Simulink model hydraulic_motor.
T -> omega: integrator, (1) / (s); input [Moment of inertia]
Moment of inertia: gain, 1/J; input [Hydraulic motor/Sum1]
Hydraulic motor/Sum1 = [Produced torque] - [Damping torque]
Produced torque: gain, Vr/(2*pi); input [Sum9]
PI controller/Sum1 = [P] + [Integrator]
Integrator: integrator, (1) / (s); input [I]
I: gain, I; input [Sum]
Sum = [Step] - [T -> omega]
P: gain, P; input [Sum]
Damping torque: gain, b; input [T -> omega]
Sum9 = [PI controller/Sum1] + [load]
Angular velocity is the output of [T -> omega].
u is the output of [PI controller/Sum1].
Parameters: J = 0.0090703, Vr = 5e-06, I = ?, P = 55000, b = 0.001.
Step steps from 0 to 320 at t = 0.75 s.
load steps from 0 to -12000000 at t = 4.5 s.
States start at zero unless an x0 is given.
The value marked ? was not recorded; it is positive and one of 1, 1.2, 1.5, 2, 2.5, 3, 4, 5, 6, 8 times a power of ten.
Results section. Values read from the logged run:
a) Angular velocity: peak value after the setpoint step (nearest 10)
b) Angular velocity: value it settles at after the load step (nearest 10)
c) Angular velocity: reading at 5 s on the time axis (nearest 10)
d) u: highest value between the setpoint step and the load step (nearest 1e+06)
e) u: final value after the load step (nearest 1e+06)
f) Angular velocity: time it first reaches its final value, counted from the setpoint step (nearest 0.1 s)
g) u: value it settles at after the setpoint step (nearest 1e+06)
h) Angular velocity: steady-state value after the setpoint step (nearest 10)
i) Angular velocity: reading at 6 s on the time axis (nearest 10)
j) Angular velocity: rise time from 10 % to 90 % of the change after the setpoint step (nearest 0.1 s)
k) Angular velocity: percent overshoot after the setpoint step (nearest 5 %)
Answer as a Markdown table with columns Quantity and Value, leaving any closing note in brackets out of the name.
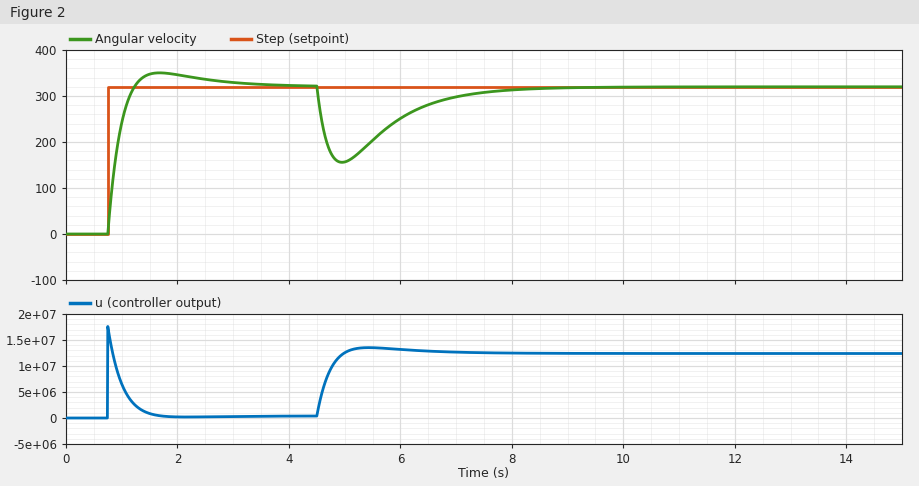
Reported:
| Quantity | Value |
|---|---|
| Angular velocity: peak value after the setpoint step | 350 |
| Angular velocity: value it settles at after the load step | 320 |
| Angular velocity: reading at 5 s on the time axis | 160 |
| u: highest value between the setpoint step and the load step | 18000000 |
| u: final value after the load step | 12000000 |
| Angular velocity: time it first reaches its final value, counted from the setpoint step | 0.5 s |
| u: value it settles at after the setpoint step | 0 |
| Angular velocity: steady-state value after the setpoint step | 320 |
| Angular velocity: reading at 6 s on the time axis | 250 |
| Angular velocity: rise time from 10 % to 90 % of the change after the setpoint step | 0.3 s |
| Angular velocity: percent overshoot after the setpoint step | 10 % |
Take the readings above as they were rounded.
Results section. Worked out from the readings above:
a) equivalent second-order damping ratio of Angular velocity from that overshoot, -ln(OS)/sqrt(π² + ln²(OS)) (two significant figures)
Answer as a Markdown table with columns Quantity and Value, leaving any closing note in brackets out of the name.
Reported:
| Quantity | Value |
|---|---|
| equivalent second-order damping ratio of Angular velocity from that overshoot, -ln(OS)/sqrt(π² + ln²(OS)) | 0.59 |
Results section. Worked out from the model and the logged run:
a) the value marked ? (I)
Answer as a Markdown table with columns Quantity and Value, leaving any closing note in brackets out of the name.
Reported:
| Quantity | Value |
|---|---|
| the value marked ? | 50000 |
